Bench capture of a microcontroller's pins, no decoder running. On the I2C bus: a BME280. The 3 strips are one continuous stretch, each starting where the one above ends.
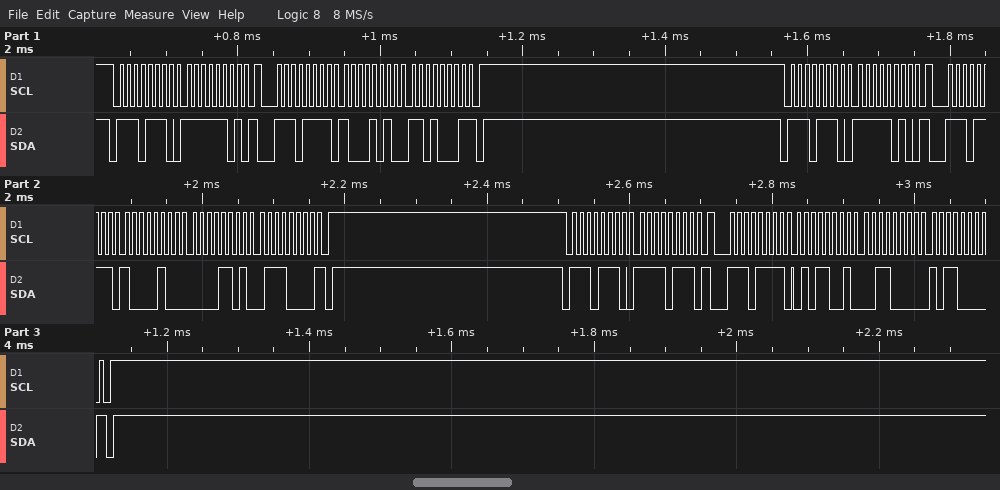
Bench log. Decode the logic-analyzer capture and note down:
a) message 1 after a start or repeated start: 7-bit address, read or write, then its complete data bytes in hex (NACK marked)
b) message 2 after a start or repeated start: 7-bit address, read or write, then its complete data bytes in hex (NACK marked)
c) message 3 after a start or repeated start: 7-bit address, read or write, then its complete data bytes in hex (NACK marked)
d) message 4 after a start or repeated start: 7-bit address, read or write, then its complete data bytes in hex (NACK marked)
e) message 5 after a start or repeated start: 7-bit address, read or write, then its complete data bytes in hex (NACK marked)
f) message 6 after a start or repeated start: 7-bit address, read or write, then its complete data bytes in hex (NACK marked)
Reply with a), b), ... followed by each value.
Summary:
a) 0x77 write: FD
b) 0x77 read: 8A D1 NACK
c) 0x77 write: FA
d) 0x77 read: 84 0D 70 NACK
e) 0x77 write: F7
f) 0x77 read: 59 30 B0 NACK
